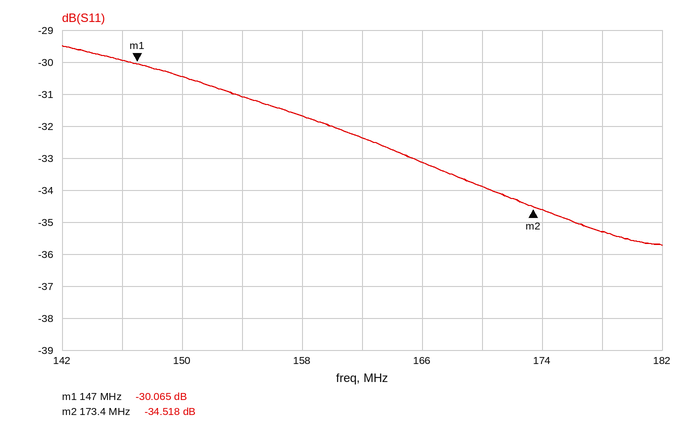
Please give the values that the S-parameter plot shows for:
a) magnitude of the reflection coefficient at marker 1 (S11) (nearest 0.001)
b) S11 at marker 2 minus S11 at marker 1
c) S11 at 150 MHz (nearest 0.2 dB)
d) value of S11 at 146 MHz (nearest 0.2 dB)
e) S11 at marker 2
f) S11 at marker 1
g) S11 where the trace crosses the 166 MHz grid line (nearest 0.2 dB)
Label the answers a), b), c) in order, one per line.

a) 0.031
b) -4.453 dB
c) -30.4 dB
d) -30.0 dB
e) -34.518 dB
f) -30.065 dB
g) -33.2 dB
